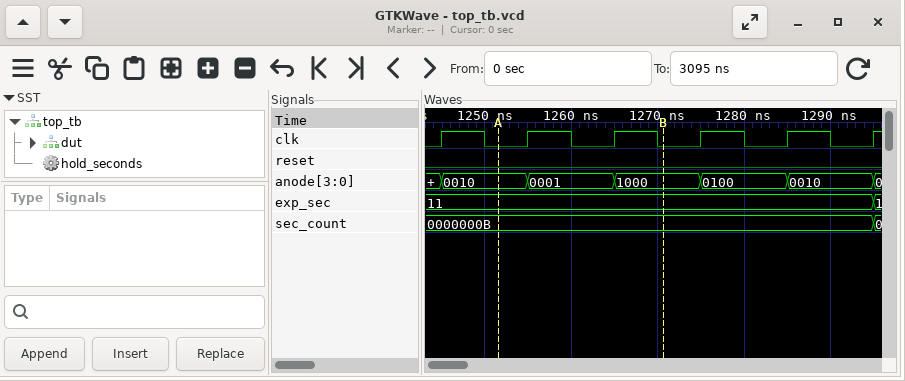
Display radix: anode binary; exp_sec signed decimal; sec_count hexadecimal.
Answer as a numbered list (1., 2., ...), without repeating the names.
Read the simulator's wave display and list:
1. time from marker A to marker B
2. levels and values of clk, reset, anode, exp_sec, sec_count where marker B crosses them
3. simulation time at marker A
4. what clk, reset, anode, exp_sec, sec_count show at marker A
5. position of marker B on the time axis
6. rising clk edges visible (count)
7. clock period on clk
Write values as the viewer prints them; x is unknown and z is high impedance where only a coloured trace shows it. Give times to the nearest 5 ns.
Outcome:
1. 20 ns
2. clk=0, reset=0, anode=1000, exp_sec=11, sec_count=0000000B
3. 1250 ns
4. clk=0, reset=0, anode=0010, exp_sec=11, sec_count=0000000B
5. 1270 ns
6. 6
7. 10 ns
